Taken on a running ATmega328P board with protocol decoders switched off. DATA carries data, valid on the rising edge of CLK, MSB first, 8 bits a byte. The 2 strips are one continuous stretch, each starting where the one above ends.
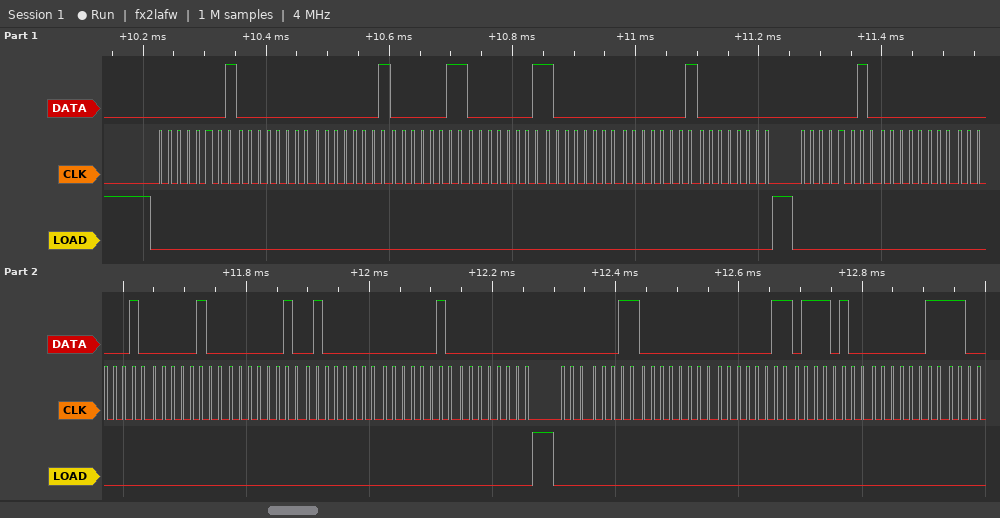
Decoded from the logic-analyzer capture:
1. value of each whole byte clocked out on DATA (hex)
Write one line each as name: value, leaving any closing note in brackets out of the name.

value of each whole byte clocked out on DATA: 01 00 01 03 01 80 01 00 02 00 02 04 02 40 02 00 03 00 03 74 03
